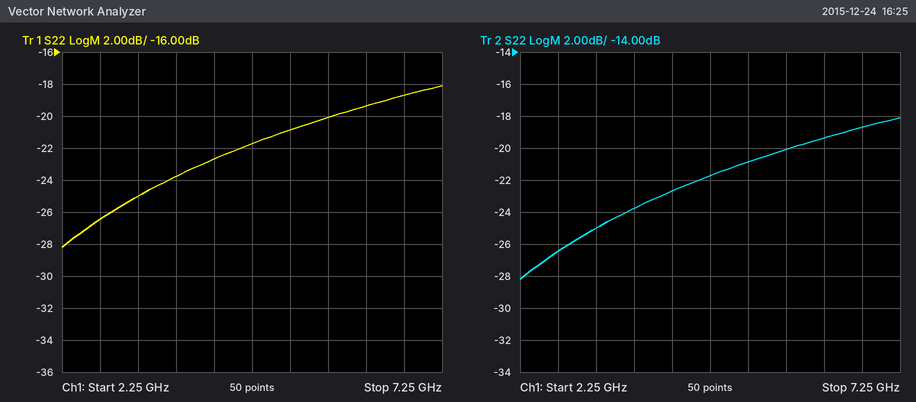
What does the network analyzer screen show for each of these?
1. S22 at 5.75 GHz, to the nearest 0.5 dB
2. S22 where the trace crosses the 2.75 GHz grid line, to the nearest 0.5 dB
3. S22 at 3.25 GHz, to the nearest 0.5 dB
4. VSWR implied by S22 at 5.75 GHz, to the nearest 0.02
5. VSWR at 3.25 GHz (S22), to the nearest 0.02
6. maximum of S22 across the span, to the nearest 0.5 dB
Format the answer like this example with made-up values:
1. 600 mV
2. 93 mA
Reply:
1. -20.0 dB
2. -26.5 dB
3. -25.0 dB
4. 1.22
5. 1.12
6. -18.0 dB
